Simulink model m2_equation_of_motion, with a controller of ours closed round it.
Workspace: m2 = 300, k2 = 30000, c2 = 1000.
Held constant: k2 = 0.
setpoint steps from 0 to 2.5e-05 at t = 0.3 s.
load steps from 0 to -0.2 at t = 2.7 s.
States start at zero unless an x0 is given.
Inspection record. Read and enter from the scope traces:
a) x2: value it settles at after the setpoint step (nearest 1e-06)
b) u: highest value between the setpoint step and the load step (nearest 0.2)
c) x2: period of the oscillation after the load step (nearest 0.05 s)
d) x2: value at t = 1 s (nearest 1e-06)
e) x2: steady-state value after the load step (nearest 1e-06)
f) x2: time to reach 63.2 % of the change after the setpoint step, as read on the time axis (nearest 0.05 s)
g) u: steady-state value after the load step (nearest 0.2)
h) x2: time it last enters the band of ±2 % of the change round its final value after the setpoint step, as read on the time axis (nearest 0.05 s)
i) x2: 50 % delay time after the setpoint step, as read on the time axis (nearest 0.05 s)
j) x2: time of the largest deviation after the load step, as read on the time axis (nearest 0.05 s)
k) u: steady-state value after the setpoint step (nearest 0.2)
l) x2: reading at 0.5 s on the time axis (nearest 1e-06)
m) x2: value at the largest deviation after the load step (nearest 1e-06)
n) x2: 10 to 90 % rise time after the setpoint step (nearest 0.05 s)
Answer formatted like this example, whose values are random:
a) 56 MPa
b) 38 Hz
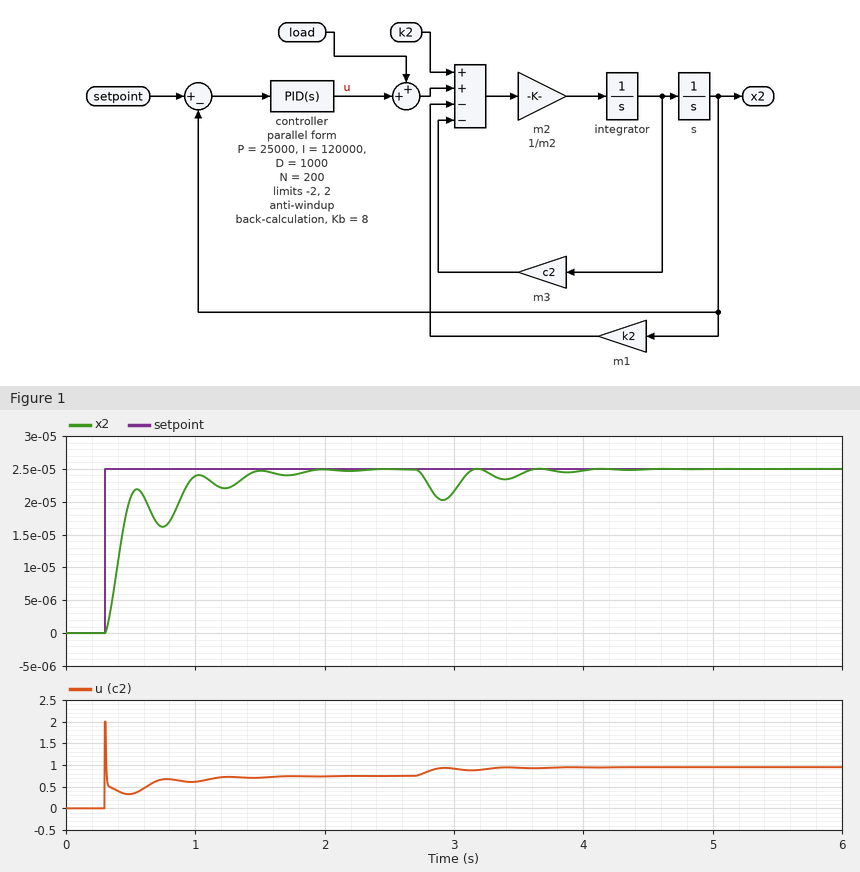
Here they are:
a) 0.000025
b) 2.0
c) 0.50 s
d) 0.000024
e) 0.000025
f) 0.45 s
g) 1.0
h) 1.85 s
i) 0.40 s
j) 2.90 s
k) 0.8
l) 0.000021
m) 0.000020
n) 0.60 s
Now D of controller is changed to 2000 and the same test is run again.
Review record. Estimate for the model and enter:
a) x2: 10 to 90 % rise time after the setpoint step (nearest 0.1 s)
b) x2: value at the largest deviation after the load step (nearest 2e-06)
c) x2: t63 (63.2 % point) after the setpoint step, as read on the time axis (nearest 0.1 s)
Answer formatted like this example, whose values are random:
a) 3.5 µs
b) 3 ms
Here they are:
a) 0.8 s
b) 0.000020
c) 0.5 s
